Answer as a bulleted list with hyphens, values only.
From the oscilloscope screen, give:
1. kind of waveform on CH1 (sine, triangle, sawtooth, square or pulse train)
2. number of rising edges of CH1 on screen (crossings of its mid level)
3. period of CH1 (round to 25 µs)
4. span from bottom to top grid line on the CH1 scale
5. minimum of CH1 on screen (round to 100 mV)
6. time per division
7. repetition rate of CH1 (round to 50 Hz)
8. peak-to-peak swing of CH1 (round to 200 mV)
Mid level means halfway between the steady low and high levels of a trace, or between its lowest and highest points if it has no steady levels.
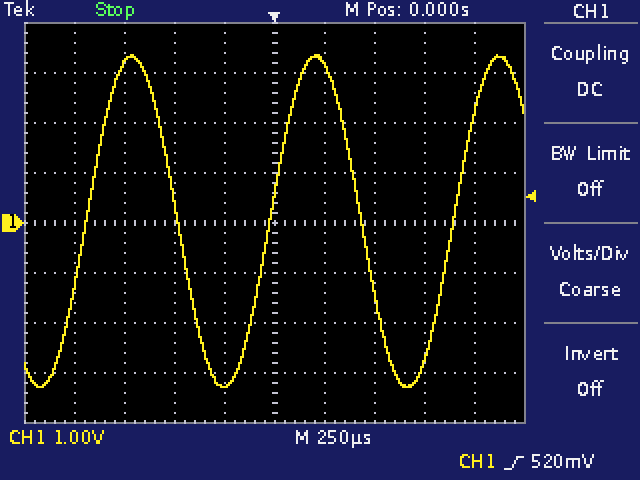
- sine
- 3
- 925 µs
- 8 V
- -3.3 V
- 250 µs
- 1.10 kHz
- 6.6 V
